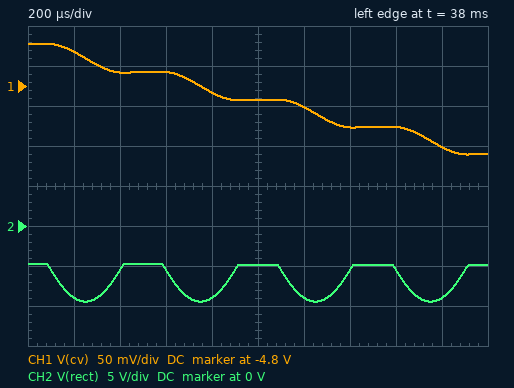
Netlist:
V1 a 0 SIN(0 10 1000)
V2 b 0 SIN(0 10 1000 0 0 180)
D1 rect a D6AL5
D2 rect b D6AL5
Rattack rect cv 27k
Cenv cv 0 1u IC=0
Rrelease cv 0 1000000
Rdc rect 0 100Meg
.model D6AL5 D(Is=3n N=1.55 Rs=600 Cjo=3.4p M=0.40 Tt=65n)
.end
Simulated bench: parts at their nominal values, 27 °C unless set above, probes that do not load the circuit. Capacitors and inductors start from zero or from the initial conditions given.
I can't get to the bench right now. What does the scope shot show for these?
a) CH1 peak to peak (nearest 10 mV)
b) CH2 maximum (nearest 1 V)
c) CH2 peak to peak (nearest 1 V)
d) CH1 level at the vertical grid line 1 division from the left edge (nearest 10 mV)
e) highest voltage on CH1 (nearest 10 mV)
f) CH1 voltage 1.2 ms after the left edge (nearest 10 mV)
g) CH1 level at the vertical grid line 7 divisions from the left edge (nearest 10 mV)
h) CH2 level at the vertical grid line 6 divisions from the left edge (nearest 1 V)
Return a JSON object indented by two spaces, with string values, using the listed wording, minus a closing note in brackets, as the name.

{
  "CH1 peak to peak": "140 mV",
  "CH2 maximum": "-5 V",
  "CH2 peak to peak": "5 V",
  "CH1 level at the vertical grid line 1 division from the left edge": "-4.76 V",
  "highest voltage on CH1": "-4.75 V",
  "CH1 voltage 1.2 ms after the left edge": "-4.83 V",
  "CH1 level at the vertical grid line 7 divisions from the left edge": "-4.85 V",
  "CH2 level at the vertical grid line 6 divisions from the left edge": "-9 V"
}
